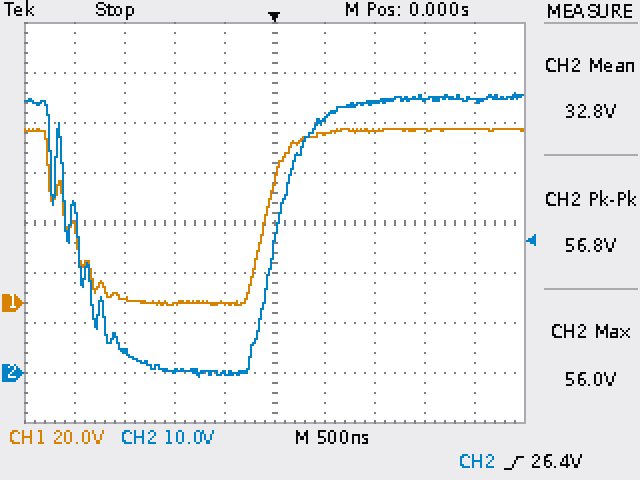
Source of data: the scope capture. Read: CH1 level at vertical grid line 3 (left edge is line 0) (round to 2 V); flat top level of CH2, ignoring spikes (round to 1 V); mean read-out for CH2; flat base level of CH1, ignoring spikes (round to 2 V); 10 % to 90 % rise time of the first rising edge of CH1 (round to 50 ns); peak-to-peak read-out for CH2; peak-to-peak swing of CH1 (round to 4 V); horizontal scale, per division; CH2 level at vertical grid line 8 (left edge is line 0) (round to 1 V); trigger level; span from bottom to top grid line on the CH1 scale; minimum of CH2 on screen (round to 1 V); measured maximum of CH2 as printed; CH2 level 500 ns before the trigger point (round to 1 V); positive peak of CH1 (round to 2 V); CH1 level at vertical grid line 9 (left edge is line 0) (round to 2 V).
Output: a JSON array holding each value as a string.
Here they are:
["0 V", "55 V", "32.8 V", "0 V", "400 ns", "56.8 V", "72 V", "500 ns", "55 V", "26.4 V", "160 V", "-1 V", "56.0 V", "0 V", "70 V", "70 V"]
